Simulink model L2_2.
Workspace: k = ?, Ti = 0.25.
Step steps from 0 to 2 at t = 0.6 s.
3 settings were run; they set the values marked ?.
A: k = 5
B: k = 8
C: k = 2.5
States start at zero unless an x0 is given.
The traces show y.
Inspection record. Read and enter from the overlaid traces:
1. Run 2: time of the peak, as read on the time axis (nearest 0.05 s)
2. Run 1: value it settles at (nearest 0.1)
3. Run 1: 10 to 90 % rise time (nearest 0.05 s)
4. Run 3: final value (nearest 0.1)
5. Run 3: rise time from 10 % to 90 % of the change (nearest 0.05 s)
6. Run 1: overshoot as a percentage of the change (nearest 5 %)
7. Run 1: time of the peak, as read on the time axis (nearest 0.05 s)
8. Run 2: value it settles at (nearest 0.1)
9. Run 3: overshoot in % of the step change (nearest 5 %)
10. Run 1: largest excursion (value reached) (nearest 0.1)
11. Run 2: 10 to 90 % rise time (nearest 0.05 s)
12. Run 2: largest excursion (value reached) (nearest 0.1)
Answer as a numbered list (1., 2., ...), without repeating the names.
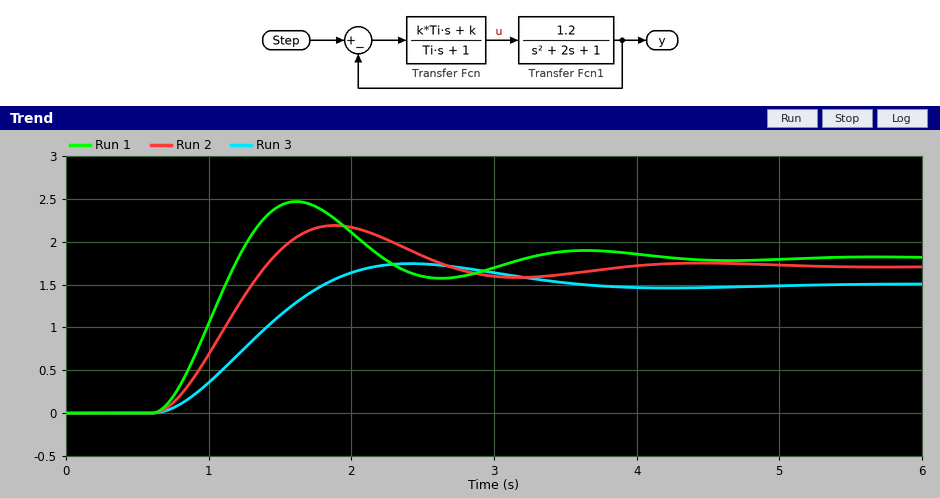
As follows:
1. 1.90 s
2. 1.8
3. 0.40 s
4. 1.5
5. 0.80 s
6. 35 %
7. 1.60 s
8. 1.7
9. 15 %
10. 2.5
11. 0.55 s
12. 2.2
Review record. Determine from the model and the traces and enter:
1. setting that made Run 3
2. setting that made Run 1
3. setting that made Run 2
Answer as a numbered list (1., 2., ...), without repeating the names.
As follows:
1. C
2. B
3. A
